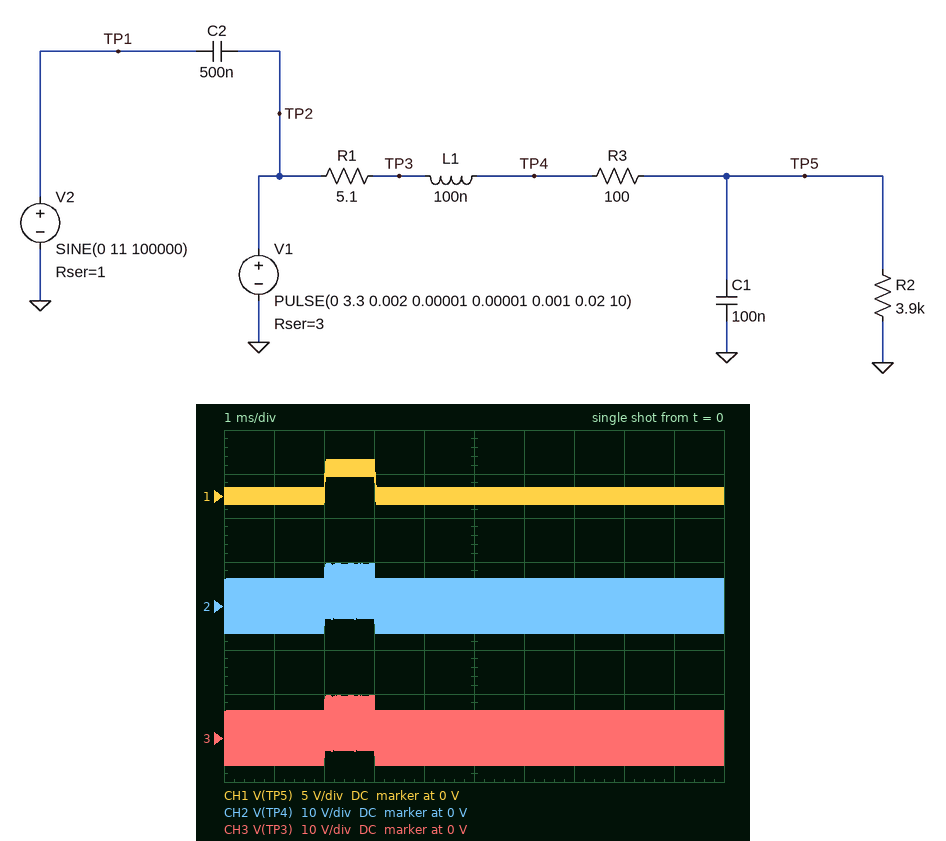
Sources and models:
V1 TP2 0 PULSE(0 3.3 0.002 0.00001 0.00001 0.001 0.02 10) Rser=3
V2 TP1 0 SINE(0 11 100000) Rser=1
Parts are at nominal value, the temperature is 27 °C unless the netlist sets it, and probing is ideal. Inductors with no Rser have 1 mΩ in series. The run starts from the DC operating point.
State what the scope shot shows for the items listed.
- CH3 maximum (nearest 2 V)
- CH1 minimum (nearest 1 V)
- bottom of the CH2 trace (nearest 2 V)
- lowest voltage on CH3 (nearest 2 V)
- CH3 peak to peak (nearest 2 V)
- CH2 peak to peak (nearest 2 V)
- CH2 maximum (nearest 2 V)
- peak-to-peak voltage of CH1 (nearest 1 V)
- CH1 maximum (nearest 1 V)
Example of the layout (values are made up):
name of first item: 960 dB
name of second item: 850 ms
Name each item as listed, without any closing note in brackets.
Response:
CH3 maximum: 10 V
CH1 minimum: -1 V
bottom of the CH2 trace: -6 V
lowest voltage on CH3: -6 V
CH3 peak to peak: 16 V
CH2 peak to peak: 16 V
CH2 maximum: 10 V
peak-to-peak voltage of CH1: 5 V
CH1 maximum: 4 V
